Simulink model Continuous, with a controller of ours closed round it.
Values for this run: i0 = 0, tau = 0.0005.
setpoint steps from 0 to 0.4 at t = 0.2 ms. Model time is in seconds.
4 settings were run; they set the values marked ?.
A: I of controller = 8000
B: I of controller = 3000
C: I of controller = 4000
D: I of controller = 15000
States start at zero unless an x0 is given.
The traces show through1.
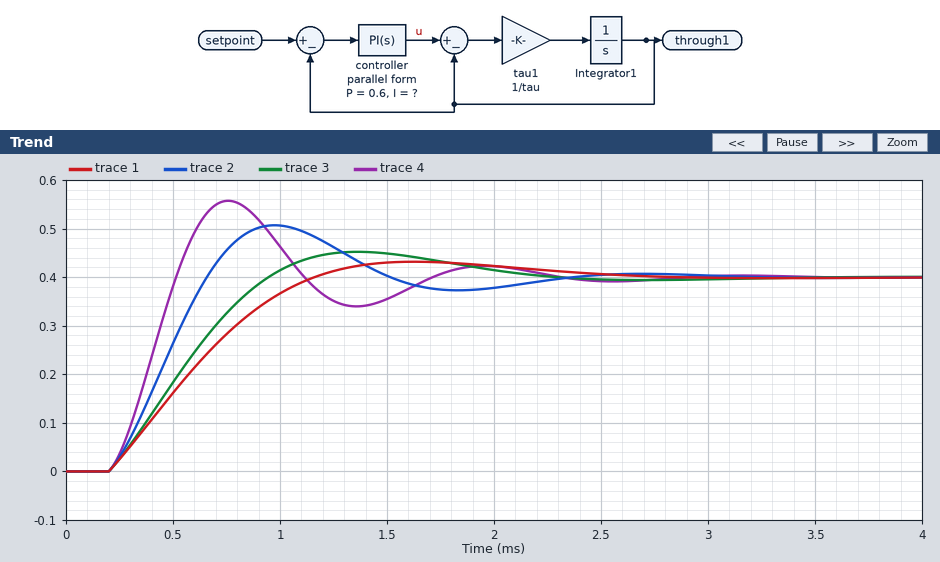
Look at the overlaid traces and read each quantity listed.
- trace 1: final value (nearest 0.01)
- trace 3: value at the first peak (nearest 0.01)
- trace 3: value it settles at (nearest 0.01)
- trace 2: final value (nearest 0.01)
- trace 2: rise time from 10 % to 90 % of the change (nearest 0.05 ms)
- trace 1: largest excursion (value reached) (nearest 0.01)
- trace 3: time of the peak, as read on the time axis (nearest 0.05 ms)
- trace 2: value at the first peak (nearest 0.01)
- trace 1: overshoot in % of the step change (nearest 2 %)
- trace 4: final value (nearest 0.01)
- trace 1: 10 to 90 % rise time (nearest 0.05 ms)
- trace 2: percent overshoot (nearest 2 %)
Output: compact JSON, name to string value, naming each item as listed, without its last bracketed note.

{"trace 1: final value": "0.40", "trace 3: value at the first peak": "0.45", "trace 3: value it settles at": "0.40", "trace 2: final value": "0.40", "trace 2: rise time from 10 % to 90 % of the change": "0.35 ms", "trace 1: largest excursion (value reached)": "0.43", "trace 3: time of the peak, as read on the time axis": "1.35 ms", "trace 2: value at the first peak": "0.51", "trace 1: overshoot in % of the step change": "8 %", "trace 4: final value": "0.40", "trace 1: 10 to 90 % rise time": "0.70 ms", "trace 2: percent overshoot": "26 %"}
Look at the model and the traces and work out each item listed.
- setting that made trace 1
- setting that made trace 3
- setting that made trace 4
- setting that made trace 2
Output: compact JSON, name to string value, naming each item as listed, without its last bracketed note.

{"setting that made trace 1": "B", "setting that made trace 3": "C", "setting that made trace 4": "D", "setting that made trace 2": "A"}
